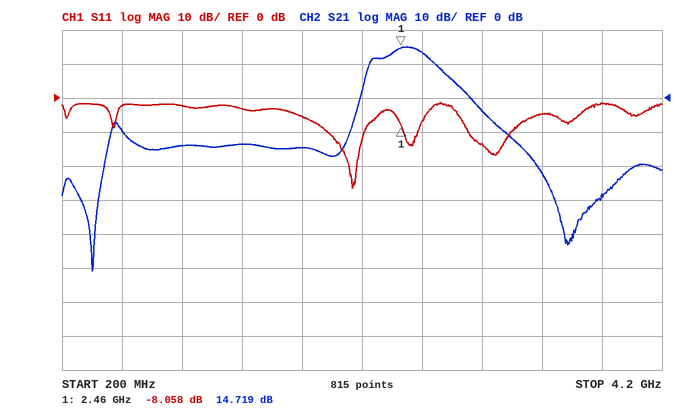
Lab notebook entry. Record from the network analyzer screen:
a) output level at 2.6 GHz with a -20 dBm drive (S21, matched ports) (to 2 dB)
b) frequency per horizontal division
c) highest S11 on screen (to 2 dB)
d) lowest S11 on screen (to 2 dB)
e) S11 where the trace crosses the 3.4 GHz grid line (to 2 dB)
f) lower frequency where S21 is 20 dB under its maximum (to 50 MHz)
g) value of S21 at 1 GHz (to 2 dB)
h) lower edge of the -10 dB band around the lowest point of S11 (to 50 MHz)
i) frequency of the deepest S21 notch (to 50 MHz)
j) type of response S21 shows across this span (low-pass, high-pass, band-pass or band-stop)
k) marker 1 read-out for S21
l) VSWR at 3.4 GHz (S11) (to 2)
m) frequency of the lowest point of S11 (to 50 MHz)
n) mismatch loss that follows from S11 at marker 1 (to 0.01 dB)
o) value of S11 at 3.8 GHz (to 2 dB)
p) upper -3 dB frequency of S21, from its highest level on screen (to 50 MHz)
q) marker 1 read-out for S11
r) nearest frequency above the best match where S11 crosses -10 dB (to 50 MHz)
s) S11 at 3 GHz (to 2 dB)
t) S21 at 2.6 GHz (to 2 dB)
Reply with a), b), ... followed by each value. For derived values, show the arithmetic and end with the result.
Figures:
a) -20 dBm + (14 dB) = -6 dBm
b) 400 MHz
c) -2 dB
d) -26 dB
e) -4 dB
f) 2.15 GHz
g) -14 dB
h) 1.95 GHz
i) 400 MHz
j) band-pass
k) 14.719 dB
l) |Γ| = 10^(-4/20) = 0.6310; VSWR = (1 + 0.6310)/(1 − 0.6310) ≈ 4
m) 2.15 GHz
n) −10 log10(1 − 10^(-8.058/10)) ≈ 0.74 dB
o) -2 dB
p) 2.65 GHz
q) -8.058 dB
r) 2.20 GHz
s) -14 dB
t) 14 dB
